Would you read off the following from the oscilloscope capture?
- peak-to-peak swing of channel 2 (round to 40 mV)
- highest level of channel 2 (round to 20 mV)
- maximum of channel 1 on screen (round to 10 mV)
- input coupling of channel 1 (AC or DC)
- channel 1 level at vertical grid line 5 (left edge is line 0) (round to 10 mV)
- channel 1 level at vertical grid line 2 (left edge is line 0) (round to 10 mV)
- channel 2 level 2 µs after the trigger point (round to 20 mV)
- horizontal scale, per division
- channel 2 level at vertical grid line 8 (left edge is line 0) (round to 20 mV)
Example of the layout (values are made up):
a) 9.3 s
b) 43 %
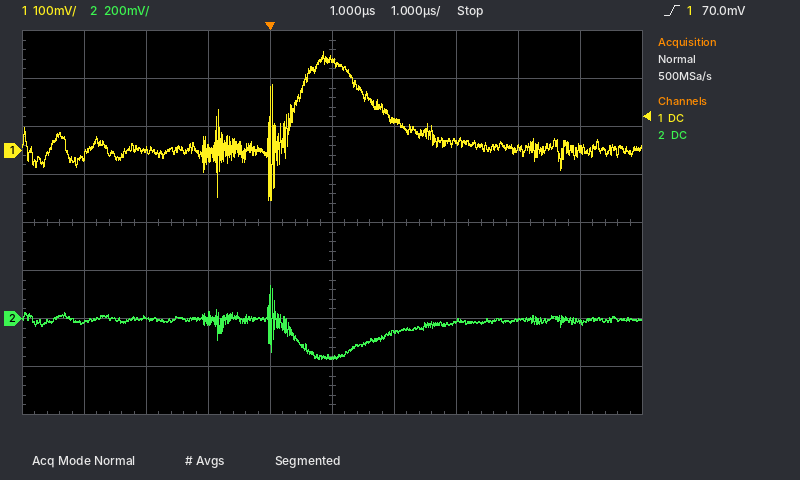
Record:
a) 320 mV
b) 140 mV
c) 210 mV
d) DC
e) 190 mV
f) 0 mV
g) -60 mV
h) 1 µs
i) 0 mV
